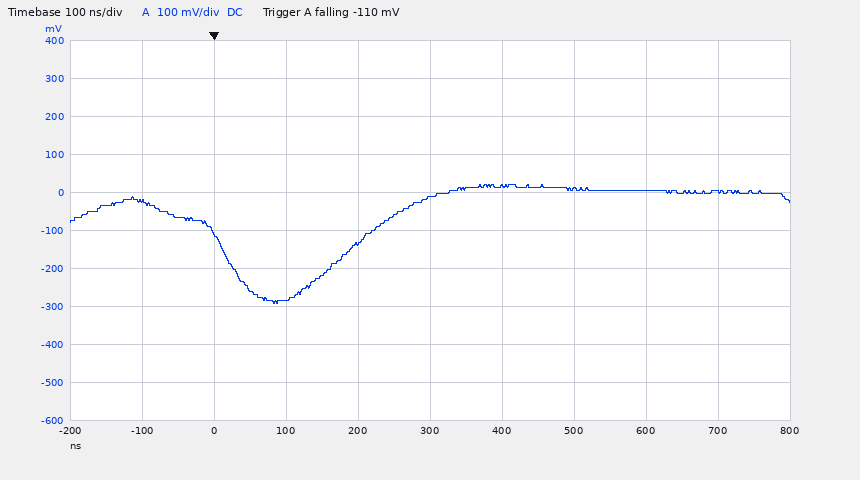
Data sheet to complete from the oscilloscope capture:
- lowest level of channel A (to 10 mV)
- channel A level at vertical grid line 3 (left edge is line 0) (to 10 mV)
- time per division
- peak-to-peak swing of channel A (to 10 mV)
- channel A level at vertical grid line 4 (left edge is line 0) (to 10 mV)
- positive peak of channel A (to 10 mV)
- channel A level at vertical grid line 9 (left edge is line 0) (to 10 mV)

-290 mV
-280 mV
100 ns
310 mV
-130 mV
20 mV
0 mV
